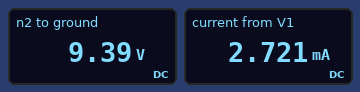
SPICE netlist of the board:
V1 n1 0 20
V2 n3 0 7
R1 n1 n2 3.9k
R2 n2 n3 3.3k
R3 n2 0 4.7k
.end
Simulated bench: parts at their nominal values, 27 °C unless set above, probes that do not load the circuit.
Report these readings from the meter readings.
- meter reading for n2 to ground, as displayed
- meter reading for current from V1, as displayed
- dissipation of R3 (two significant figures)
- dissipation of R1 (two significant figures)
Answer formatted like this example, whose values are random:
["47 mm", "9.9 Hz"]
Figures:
["9.39 V", "2.721 mA", "19 mW", "29 mW"]
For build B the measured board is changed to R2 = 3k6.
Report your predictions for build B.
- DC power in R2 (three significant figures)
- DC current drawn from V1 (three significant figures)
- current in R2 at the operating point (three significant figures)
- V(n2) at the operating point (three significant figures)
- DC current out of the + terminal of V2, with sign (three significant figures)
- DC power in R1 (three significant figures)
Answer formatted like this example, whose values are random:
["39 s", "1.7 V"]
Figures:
["1.69 mW", "2.70 mA", "686 µA", "9.47 V", "-686 µA", "28.4 mW"]
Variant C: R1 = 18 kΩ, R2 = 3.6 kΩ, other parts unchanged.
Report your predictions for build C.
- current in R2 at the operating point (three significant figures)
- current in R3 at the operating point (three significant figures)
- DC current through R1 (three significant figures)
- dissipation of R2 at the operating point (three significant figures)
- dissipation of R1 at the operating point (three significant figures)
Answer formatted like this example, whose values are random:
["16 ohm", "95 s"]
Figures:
["390 µA", "1.19 mA", "800 µA", "548 µW", "11.5 mW"]
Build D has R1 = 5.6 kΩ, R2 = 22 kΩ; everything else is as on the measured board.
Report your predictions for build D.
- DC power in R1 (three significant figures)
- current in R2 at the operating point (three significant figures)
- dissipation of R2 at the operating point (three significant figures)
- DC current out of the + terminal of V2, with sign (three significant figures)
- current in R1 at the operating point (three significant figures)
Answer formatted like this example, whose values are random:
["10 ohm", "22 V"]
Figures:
["22.0 mW", "86.6 µA", "165 µW", "-86.6 µA", "1.98 mA"]
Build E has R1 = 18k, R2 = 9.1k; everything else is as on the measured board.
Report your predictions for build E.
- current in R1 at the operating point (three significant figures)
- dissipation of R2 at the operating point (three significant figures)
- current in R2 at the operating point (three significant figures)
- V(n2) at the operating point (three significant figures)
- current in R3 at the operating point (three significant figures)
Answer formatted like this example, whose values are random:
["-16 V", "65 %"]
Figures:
["835 µA", "452 µW", "223 µA", "4.97 V", "1.06 mA"]
